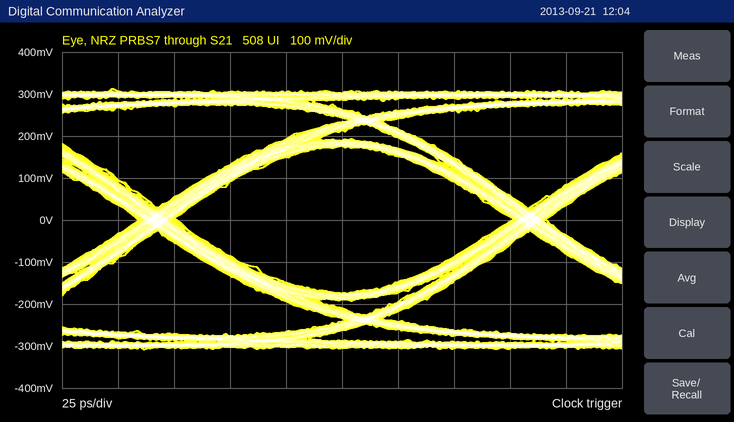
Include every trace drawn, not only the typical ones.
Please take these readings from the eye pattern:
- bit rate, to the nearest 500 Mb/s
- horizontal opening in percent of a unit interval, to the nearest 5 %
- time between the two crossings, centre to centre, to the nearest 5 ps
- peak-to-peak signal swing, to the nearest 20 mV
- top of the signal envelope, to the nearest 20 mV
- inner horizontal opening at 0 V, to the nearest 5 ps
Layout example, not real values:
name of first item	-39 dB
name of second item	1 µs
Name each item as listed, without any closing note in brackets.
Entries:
bit rate, to the nearest 500 Mb/s	6.0 Gb/s
horizontal opening in percent of a unit interval, to the nearest 5 %	90 %
time between the two crossings, centre to centre, to the nearest 5 ps	165 ps
peak-to-peak signal swing, to the nearest 20 mV	620 mV
top of the signal envelope, to the nearest 20 mV	320 mV
inner horizontal opening at 0 V, to the nearest 5 ps	150 ps
